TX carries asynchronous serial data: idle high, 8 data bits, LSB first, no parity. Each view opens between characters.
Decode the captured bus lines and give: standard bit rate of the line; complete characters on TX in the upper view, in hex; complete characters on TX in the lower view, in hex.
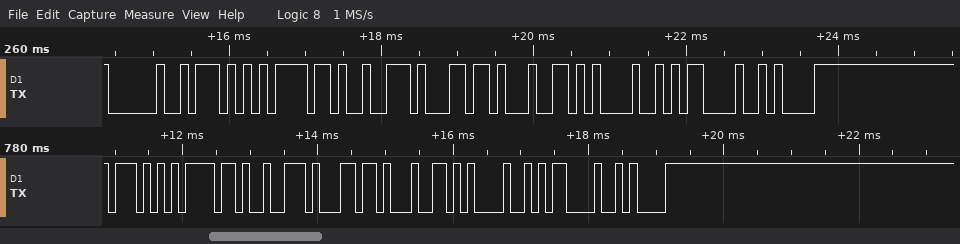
9600 baud
20, 57, 6F, 72, 6C, 64, 21, 0D, 0A
57, 6F, 72, 6C, 64, 21, 0D, 0A
